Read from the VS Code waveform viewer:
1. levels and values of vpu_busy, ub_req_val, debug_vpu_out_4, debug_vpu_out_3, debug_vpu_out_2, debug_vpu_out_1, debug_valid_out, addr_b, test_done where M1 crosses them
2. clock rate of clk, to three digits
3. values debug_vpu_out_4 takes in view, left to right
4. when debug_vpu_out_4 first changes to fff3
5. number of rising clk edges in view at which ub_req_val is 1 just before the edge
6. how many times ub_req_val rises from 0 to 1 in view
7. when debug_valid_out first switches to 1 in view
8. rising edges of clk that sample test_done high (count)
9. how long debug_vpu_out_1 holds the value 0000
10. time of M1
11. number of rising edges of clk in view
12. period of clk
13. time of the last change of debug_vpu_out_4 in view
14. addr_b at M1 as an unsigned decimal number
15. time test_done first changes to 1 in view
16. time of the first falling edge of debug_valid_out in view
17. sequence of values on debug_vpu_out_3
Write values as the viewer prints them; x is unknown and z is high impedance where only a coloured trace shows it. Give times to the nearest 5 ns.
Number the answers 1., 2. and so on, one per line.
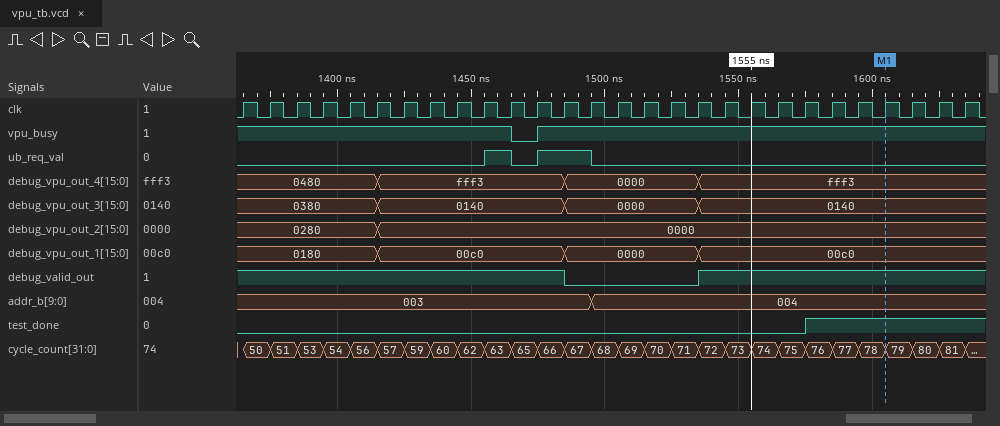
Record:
1. vpu_busy=1, ub_req_val=0, debug_vpu_out_4=fff3, debug_vpu_out_3=0140, debug_vpu_out_2=0000, debug_vpu_out_1=00c0, debug_valid_out=1, addr_b=004, test_done=1
2. 100 MHz
3. 0480, fff3, 0000, fff3
4. 1415 ns
5. 3
6. 2
7. 1535 ns
8. 6
9. 50 ns
10. 1605 ns
11. 28
12. 10 ns
13. 1535 ns
14. 4
15. 1575 ns
16. 1485 ns
17. 0380, 0140, 0000, 0140
